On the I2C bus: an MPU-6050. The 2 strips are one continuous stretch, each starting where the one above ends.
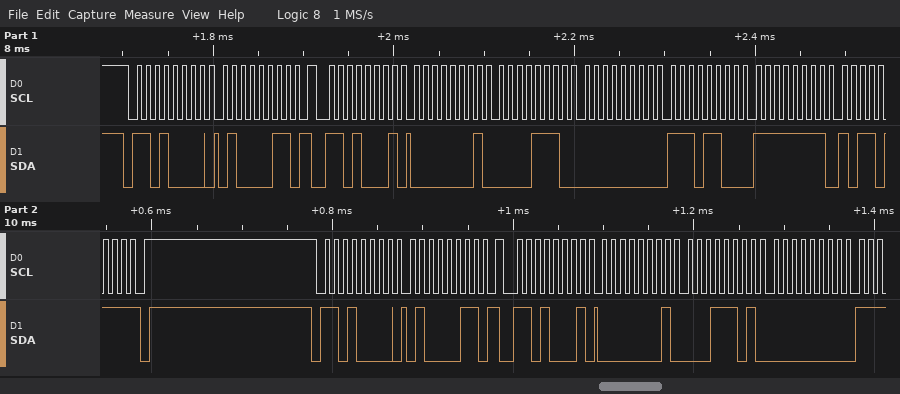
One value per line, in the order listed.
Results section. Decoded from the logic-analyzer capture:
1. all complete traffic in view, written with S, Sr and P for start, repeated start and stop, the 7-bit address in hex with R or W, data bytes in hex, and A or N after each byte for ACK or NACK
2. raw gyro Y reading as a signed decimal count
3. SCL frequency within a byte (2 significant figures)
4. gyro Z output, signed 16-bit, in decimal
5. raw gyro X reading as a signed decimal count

S 68W A 43 A Sr 68R A 01 A 0E A 00 A EC A FF A B7 N P S 68W A 43 A Sr 68R A 01 A 1D A 00 A
236
100 kHz
-73
270
